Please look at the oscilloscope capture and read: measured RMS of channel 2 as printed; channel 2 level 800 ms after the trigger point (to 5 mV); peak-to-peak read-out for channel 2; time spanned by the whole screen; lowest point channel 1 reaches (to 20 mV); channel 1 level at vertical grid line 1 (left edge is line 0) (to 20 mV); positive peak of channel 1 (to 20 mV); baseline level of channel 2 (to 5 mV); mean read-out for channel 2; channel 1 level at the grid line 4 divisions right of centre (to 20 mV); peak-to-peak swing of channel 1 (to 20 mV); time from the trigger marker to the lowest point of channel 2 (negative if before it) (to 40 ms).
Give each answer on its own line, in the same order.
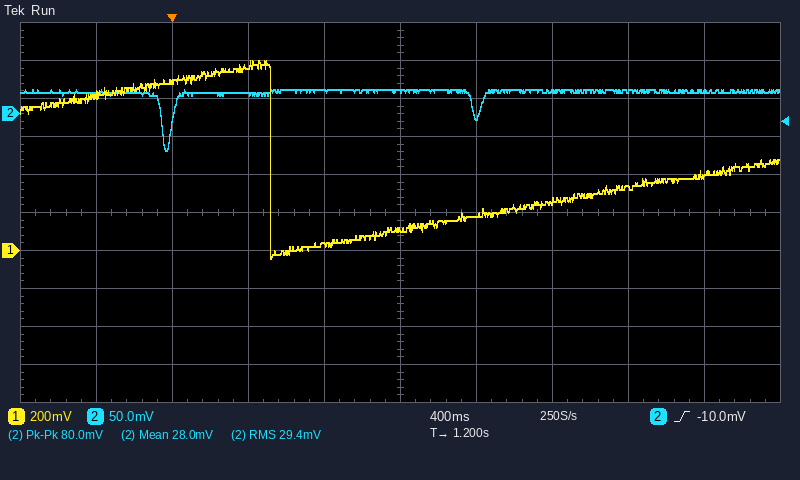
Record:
29.4 mV
30 mV
80.0 mV
4 s
-40 mV
820 mV
1.00 V
30 mV
28.0 mV
400 mV
1.04 V
-40 ms
